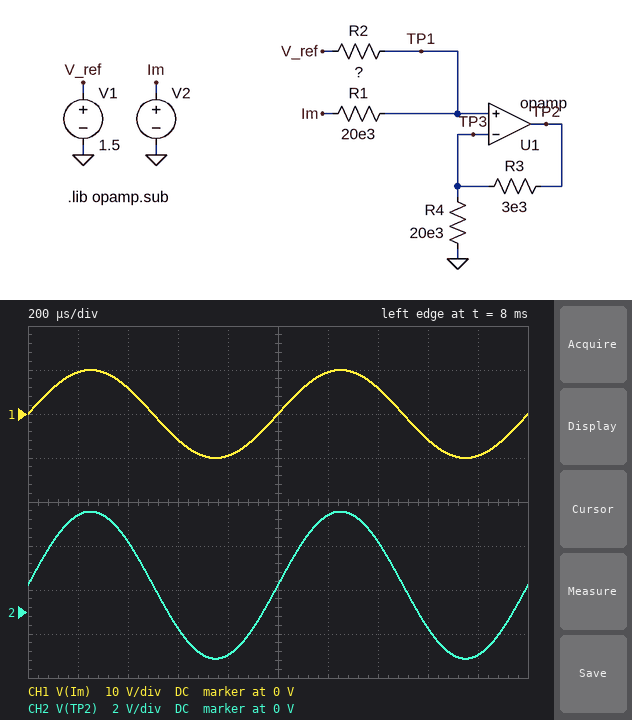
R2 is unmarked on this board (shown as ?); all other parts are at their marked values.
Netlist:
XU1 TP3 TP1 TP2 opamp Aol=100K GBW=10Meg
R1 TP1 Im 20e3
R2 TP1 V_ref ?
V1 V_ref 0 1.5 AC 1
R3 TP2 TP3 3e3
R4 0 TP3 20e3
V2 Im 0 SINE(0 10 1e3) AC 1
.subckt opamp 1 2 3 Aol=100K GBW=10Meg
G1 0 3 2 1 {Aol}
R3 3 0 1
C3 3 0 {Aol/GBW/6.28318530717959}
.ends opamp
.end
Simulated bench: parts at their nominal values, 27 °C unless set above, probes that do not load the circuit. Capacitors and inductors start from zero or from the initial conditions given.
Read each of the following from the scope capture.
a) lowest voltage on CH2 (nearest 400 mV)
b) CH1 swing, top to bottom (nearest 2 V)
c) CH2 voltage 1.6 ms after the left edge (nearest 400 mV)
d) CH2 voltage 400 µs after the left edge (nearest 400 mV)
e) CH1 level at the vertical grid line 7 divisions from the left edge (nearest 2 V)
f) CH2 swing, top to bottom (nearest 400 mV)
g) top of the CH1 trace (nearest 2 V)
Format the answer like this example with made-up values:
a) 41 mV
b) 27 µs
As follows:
a) -2.0 V
b) 20 V
c) -800 mV
d) 3.2 V
e) 6 V
f) 6.8 V
g) 10 V
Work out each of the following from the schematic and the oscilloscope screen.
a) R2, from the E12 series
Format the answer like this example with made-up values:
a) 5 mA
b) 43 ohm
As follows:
a) 8.2 kΩ
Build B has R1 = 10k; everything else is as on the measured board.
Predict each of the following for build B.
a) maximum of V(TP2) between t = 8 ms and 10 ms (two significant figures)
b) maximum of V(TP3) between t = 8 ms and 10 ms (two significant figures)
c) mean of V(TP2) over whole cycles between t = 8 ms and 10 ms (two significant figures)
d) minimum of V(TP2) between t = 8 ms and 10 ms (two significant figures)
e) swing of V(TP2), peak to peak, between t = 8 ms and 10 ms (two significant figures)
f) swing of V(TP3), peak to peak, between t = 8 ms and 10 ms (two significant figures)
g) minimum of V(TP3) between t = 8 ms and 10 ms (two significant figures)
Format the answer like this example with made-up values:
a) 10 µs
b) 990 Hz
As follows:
a) 6.1 V
b) 5.3 V
c) 950 mV
d) -4.2 V
e) 10 V
f) 9.0 V
g) -3.7 V
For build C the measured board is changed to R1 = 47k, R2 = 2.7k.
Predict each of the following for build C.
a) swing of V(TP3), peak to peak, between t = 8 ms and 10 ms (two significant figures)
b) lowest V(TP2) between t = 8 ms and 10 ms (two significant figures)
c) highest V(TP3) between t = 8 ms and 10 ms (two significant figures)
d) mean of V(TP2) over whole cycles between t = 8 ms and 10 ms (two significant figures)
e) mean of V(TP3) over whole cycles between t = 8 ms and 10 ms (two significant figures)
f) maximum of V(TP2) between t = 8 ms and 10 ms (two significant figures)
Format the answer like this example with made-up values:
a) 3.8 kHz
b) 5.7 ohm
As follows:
a) 1.1 V
b) 1.0 V
c) 2.0 V
d) 1.6 V
e) 1.4 V
f) 2.3 V
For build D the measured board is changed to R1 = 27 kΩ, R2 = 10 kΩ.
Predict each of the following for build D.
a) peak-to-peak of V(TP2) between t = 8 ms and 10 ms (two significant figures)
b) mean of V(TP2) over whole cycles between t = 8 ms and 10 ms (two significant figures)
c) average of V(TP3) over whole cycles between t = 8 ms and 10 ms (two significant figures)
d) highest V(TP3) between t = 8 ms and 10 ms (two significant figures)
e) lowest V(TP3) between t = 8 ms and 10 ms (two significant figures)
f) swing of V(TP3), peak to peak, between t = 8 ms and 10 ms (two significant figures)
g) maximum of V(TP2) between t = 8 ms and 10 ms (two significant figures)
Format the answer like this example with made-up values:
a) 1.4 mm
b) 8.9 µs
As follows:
a) 6.2 V
b) 1.3 V
c) 1.1 V
d) 3.8 V
e) -1.6 V
f) 5.4 V
g) 4.4 V
